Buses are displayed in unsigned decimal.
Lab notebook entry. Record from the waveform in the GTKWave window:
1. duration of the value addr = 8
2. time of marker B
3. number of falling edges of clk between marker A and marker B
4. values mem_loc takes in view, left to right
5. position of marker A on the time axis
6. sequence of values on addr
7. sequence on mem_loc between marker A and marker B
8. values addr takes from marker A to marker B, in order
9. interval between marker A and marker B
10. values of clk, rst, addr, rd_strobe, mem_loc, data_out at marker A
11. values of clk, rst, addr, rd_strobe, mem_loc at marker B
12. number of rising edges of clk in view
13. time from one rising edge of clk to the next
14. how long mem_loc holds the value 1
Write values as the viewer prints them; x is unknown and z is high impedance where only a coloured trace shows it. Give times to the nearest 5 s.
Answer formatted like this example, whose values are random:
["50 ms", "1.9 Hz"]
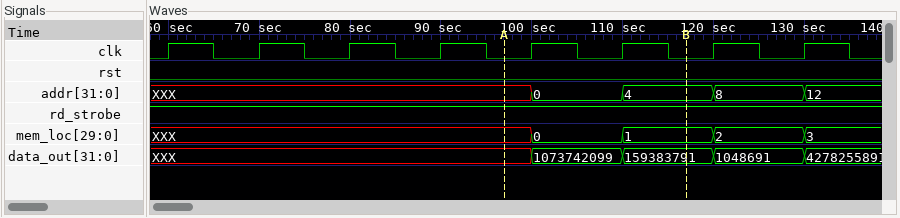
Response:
["10 s", "115 s", "2", "XXX, 0, 1, 2, 3", "95 s", "XXX, 0, 4, 8, 12", "XXX, 0, 1", "XXX, 0, 4", "20 s", "clk=0, rst=0, addr=XXX, rd_strobe=1, mem_loc=XXX, data_out=XXX", "clk=0, rst=0, addr=4, rd_strobe=1, mem_loc=1", "8", "10 s", "10 s"]
